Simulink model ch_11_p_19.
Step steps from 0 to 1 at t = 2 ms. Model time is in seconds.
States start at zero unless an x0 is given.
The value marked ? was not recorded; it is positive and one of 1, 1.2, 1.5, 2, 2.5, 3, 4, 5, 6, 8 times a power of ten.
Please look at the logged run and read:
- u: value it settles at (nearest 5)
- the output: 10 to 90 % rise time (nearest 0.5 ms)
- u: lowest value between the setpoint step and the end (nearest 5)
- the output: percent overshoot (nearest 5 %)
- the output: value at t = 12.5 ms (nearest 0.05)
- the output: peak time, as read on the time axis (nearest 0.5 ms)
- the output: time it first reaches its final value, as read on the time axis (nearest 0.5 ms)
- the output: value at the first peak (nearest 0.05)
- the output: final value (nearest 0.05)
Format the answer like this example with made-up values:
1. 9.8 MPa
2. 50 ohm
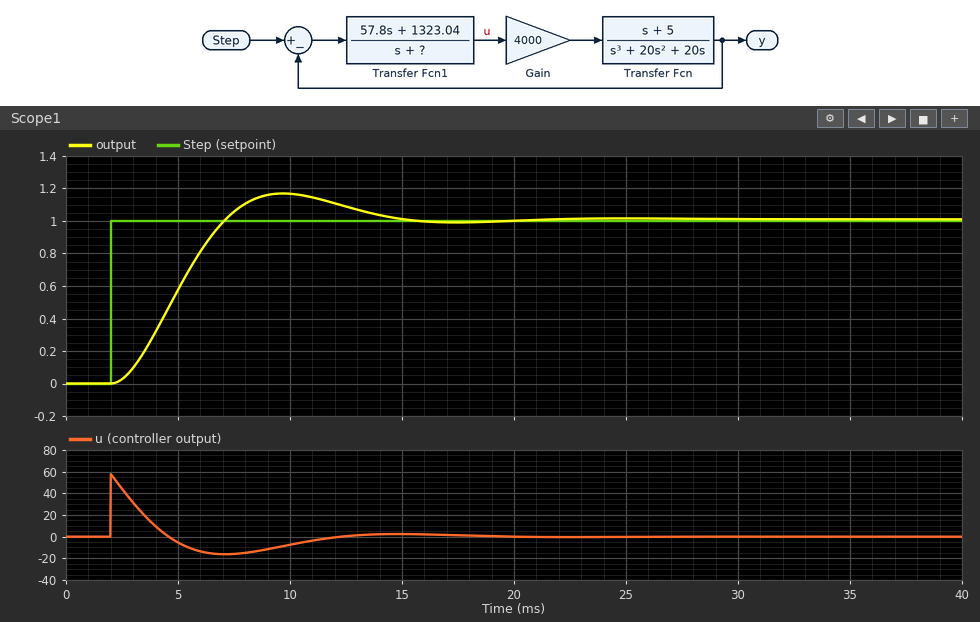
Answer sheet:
1. 0
2. 3.5 ms
3. -15
4. 15 %
5. 1.10
6. 9.5 ms
7. 7.0 ms
8. 1.15
9. 1.00
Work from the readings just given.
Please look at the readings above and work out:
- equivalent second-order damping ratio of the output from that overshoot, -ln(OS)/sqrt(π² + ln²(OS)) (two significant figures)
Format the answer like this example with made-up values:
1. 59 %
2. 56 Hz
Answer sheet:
1. 0.52
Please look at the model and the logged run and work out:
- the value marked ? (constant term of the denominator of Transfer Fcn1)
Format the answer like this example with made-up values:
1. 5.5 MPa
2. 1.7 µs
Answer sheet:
1. 500
